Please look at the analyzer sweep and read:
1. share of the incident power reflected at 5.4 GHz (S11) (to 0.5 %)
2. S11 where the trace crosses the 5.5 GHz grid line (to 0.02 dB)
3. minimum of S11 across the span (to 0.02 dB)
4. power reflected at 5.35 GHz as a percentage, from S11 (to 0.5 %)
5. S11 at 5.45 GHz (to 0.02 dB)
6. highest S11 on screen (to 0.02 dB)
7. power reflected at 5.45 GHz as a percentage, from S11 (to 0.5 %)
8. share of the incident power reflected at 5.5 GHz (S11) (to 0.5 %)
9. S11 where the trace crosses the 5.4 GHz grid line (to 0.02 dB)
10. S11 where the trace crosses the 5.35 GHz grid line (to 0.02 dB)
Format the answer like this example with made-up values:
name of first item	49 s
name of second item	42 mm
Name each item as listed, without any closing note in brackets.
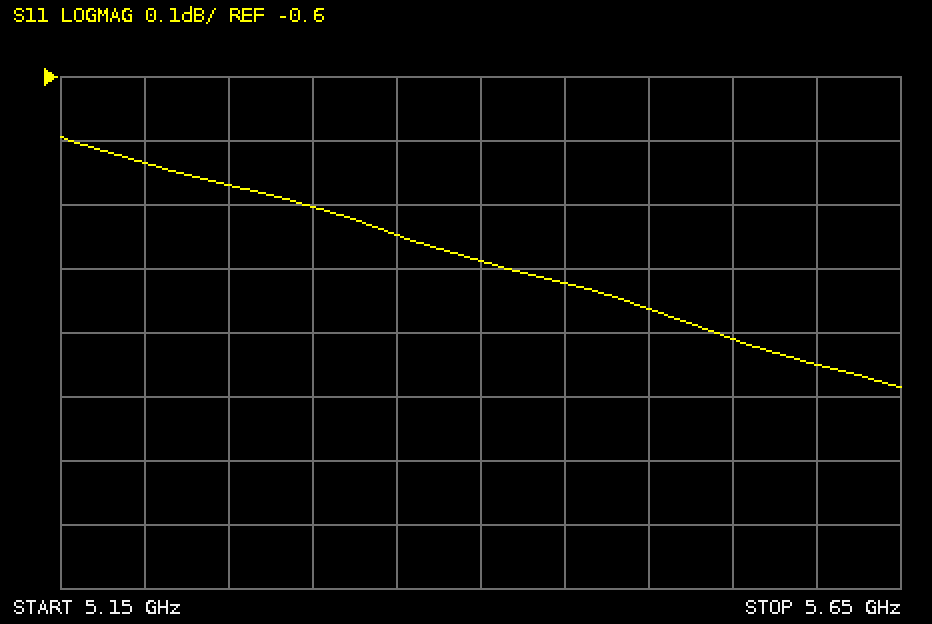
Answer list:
share of the incident power reflected at 5.4 GHz (S11)	81.5 %
S11 where the trace crosses the 5.5 GHz grid line	-0.96 dB
minimum of S11 across the span	-1.08 dB
power reflected at 5.35 GHz as a percentage, from S11	82.5 %
S11 at 5.45 GHz	-0.92 dB
highest S11 on screen	-0.70 dB
power reflected at 5.45 GHz as a percentage, from S11	81.0 %
share of the incident power reflected at 5.5 GHz (S11)	80.0 %
S11 where the trace crosses the 5.4 GHz grid line	-0.88 dB
S11 where the trace crosses the 5.35 GHz grid line	-0.84 dB
